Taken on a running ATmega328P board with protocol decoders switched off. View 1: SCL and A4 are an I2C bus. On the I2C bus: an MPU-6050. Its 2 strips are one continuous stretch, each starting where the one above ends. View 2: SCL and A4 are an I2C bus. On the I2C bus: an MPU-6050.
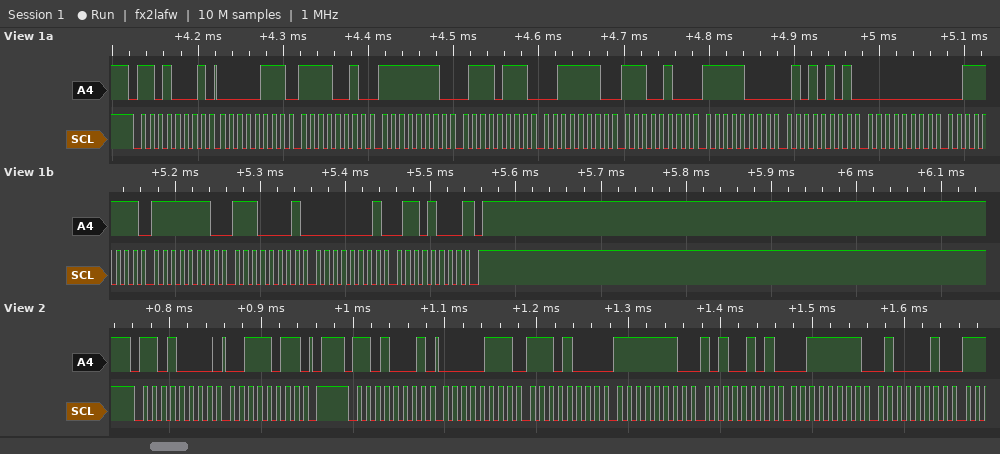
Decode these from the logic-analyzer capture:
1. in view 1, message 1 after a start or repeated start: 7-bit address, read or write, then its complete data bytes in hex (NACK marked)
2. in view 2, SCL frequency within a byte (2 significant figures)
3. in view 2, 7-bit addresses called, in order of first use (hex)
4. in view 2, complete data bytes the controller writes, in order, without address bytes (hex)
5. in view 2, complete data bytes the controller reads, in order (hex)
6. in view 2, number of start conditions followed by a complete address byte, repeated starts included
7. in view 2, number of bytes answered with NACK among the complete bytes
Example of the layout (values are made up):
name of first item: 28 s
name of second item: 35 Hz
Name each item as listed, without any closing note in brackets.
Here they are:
in view 1, message 1 after a start or repeated start: 7-bit address, read or write, then its complete data bytes in hex: 0x68 read: 07 F2 FE 77 3E E4 F8 55 00 3F FE E1 01 68 NACK
in view 2, SCL frequency within a byte: 100 kHz
in view 2, 7-bit addresses called, in order of first use: 0x68
in view 2, complete data bytes the controller writes, in order, without address bytes: 3B
in view 2, complete data bytes the controller reads, in order: 07 E8 FE A5 3F 42
in view 2, number of start conditions followed by a complete address byte, repeated starts included: 2
in view 2, number of bytes answered with NACK among the complete bytes: 0
